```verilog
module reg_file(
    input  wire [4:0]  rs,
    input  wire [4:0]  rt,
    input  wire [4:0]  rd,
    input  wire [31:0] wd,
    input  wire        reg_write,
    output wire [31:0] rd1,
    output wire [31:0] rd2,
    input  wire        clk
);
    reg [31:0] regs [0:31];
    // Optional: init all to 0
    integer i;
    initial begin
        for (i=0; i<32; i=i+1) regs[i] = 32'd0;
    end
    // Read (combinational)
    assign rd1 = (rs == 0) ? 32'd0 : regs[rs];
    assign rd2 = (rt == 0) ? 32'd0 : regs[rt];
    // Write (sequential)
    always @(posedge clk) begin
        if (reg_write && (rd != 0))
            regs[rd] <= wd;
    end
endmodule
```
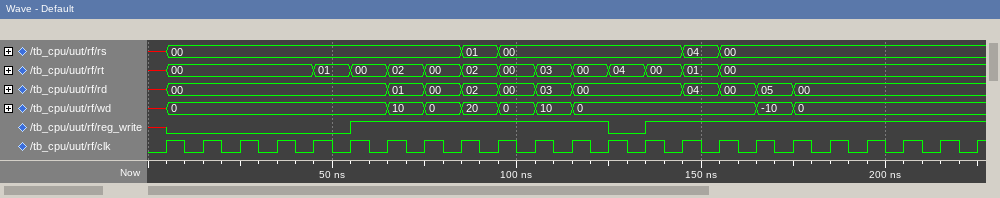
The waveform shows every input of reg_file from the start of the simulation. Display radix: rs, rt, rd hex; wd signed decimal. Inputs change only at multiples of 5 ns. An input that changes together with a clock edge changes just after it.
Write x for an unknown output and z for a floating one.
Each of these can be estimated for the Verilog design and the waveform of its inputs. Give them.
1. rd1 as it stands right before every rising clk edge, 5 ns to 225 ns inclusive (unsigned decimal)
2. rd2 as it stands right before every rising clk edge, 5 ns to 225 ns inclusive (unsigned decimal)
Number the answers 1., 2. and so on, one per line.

1. x, 0, 0, 0, 0, 0, 0, 0, 0, 10, 0, 0, 0, 0, 0, 0, 0, 0, 0, 0, 0, 0, 0
2. x, 0, 0, 0, 0, 0, 0, 0, 0, 0, 0, 0, 0, 0, 0, 10, 0, 0, 0, 0, 0, 0, 0
